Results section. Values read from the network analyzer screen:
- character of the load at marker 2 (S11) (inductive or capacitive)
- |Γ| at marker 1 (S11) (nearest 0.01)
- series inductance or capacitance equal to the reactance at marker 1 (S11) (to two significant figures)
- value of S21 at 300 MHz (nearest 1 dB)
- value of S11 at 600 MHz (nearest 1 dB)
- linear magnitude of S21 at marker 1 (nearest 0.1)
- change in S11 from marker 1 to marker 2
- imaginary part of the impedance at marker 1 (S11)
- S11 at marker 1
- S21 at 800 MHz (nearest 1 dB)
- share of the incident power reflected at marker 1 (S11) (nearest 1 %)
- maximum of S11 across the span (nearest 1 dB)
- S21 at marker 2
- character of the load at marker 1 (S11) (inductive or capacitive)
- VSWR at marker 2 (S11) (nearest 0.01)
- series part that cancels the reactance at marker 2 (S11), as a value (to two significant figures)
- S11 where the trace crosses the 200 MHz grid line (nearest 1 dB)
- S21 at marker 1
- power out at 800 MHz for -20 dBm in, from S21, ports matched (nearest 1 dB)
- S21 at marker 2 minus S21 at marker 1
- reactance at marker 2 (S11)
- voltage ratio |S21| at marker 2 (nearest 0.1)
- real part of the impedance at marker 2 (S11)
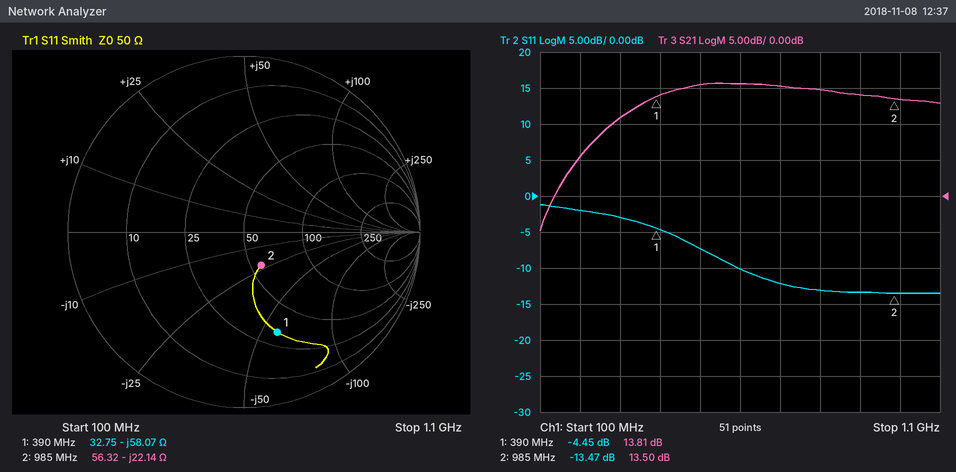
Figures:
capacitive
0.60
7.0 pF
11 dB
-10 dB
4.9
-9.02 dB
-58.07 Ω
-4.45 dB
15 dB
36 %
-1 dB
13.50 dB
capacitive
1.54
3.6 nH
-2 dB
13.81 dB
-5 dBm
-0.31 dB
-22.14 Ω
4.7
56.32 Ω
